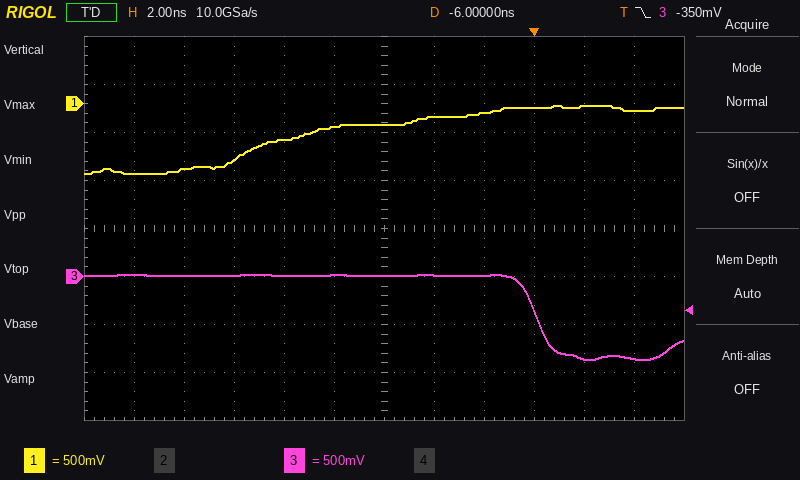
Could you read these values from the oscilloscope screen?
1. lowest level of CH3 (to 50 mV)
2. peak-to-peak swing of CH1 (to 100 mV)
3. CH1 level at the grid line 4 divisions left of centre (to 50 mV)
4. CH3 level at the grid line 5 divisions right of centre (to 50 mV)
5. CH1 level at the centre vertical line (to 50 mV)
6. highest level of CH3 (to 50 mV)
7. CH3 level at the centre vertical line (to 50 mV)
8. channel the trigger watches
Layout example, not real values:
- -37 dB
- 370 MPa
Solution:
- -850 mV
- 700 mV
- -700 mV
- -850 mV
- -200 mV
- 0 mV
- 0 mV
- CH3
